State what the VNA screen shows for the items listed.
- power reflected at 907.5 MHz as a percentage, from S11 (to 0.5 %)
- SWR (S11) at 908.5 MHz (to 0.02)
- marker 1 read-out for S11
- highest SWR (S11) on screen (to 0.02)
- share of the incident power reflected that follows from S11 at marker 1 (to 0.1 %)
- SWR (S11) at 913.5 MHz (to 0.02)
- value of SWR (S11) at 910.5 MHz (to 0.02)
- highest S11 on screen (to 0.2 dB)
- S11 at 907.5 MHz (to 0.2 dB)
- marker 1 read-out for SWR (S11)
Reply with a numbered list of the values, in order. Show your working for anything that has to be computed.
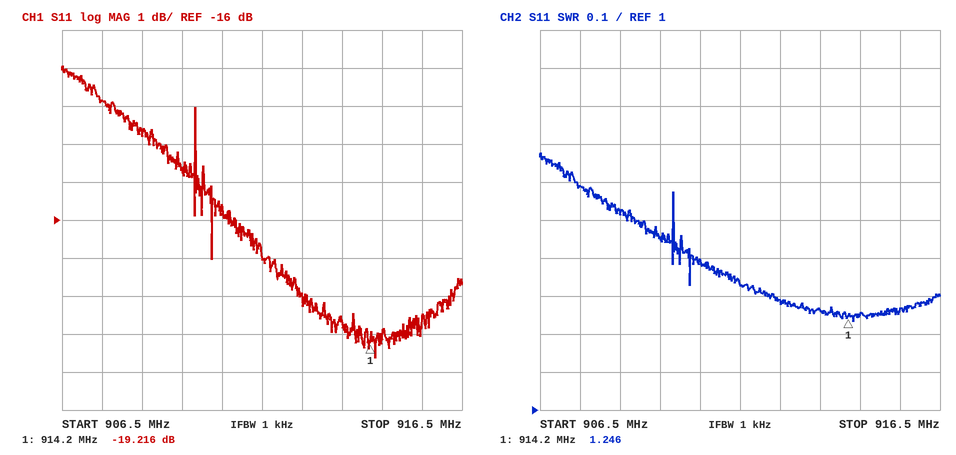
1. 10^(-12.8/10) ≈ 5.25 %, so 5.0 % to the nearest 0.5 %
2. 1.52
3. -19.216 dB
4. 1.68
5. 10^(-19.216/10) ≈ 1.2 %
6. 1.26
7. 1.40
8. -12.0 dB
9. -12.8 dB
10. 1.246
